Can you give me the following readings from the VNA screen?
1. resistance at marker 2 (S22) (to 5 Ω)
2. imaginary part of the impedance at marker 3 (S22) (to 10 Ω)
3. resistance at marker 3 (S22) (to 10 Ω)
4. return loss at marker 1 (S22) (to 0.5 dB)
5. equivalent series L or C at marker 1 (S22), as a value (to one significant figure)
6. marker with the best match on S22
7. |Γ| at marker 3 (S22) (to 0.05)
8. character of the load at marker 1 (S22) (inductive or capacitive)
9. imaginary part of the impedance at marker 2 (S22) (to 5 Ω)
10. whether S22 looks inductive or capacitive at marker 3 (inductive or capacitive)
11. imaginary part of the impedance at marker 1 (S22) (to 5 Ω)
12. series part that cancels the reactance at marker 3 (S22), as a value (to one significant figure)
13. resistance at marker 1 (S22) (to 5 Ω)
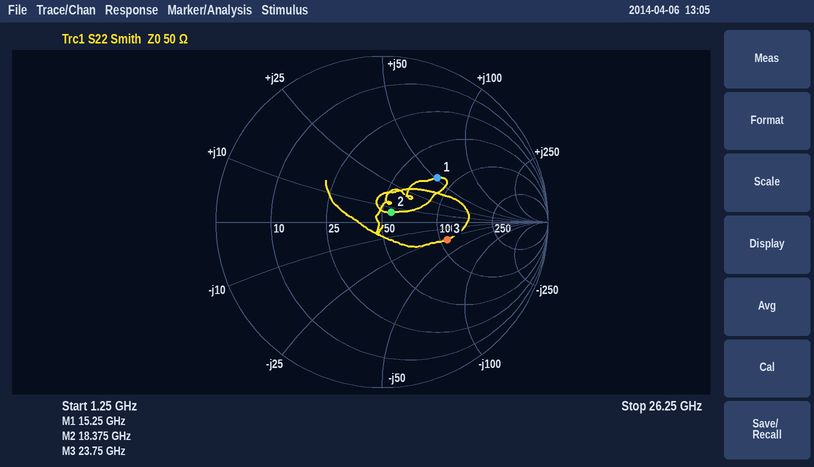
55 Ω
-30 Ω
110 Ω
7.5 dB
500 pH
marker 2
0.40
inductive
+5 Ω
capacitive
+50 Ω
200 pH
80 Ω
